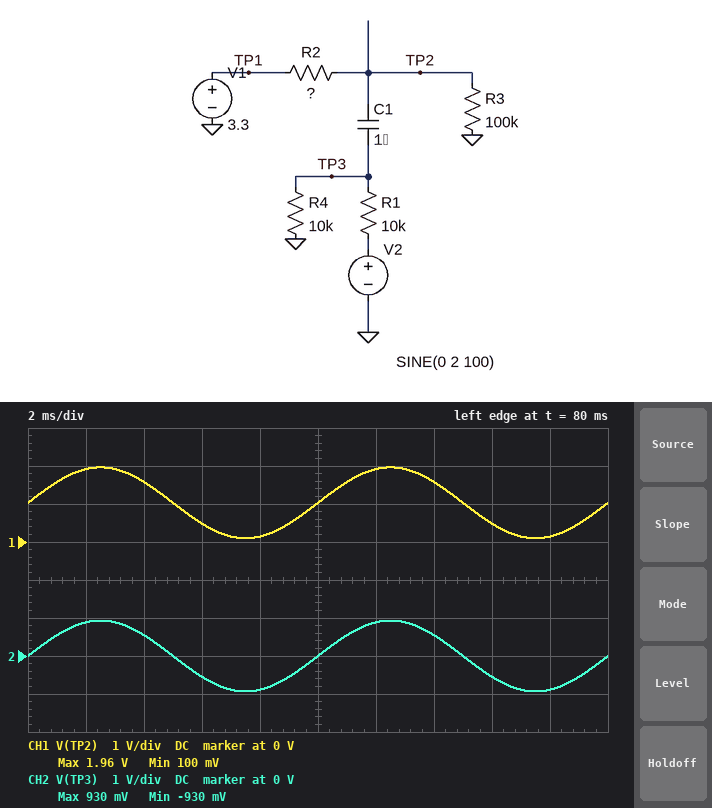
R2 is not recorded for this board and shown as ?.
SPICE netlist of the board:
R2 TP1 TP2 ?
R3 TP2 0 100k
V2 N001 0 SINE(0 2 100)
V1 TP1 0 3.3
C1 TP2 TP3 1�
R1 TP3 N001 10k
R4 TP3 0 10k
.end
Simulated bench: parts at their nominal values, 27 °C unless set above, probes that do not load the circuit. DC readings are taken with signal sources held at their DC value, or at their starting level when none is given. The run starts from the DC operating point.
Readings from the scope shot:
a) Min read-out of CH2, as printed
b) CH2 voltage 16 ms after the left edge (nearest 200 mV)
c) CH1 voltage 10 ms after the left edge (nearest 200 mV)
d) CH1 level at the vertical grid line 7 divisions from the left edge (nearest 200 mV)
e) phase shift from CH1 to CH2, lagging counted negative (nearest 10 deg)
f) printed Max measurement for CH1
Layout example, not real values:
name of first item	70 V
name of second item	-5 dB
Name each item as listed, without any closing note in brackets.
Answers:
Min read-out of CH2, as printed	-930 mV
CH2 voltage 16 ms after the left edge	-600 mV
CH1 voltage 10 ms after the left edge	1.0 V
CH1 level at the vertical grid line 7 divisions from the left edge	1.6 V
phase shift from CH1 to CH2, lagging counted negative	0 deg
printed Max measurement for CH1	1.96 V
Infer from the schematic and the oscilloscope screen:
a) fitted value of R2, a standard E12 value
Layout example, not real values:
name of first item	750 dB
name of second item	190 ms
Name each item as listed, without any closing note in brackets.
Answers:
fitted value of R2, a standard E12 value	220 kΩ
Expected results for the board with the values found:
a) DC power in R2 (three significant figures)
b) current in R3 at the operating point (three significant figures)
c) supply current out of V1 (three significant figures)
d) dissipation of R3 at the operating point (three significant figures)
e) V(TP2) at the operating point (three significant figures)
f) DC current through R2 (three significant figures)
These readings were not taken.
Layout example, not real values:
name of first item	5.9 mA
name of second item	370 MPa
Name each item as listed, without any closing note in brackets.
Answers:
DC power in R2	23.4 µW
current in R3 at the operating point	10.3 µA
supply current out of V1	10.3 µA
dissipation of R3 at the operating point	10.6 µW
V(TP2) at the operating point	1.03 V
DC current through R2	10.3 µA
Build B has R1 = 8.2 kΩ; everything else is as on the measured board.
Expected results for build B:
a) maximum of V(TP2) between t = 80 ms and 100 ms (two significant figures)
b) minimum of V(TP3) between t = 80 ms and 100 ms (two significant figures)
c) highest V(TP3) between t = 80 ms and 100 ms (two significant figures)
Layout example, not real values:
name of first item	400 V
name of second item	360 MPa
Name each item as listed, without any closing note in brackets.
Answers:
maximum of V(TP2) between t = 80 ms and 100 ms	2.1 V
minimum of V(TP3) between t = 80 ms and 100 ms	-1.0 V
highest V(TP3) between t = 80 ms and 100 ms	1.0 V
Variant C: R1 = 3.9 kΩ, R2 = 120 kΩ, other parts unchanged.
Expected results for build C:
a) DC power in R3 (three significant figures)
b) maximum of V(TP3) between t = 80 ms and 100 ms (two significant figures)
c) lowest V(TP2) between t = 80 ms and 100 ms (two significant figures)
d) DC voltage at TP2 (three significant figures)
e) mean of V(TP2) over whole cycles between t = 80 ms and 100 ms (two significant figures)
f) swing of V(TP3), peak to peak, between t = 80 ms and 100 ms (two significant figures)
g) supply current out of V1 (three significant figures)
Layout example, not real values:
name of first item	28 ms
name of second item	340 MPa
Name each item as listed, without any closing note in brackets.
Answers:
DC power in R3	22.5 µW
maximum of V(TP3) between t = 80 ms and 100 ms	1.4 V
lowest V(TP2) between t = 80 ms and 100 ms	130 mV
DC voltage at TP2	1.50 V
mean of V(TP2) over whole cycles between t = 80 ms and 100 ms	1.5 V
swing of V(TP3), peak to peak, between t = 80 ms and 100 ms	2.7 V
supply current out of V1	15.0 µA
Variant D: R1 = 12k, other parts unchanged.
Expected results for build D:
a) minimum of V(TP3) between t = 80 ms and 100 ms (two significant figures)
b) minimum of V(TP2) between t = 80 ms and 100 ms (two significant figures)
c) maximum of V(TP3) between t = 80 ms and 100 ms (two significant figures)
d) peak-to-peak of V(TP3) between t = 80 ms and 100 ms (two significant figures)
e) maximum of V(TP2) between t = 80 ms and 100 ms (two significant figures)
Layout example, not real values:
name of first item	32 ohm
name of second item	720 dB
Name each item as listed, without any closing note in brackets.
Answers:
minimum of V(TP3) between t = 80 ms and 100 ms	-840 mV
minimum of V(TP2) between t = 80 ms and 100 ms	190 mV
maximum of V(TP3) between t = 80 ms and 100 ms	840 mV
peak-to-peak of V(TP3) between t = 80 ms and 100 ms	1.7 V
maximum of V(TP2) between t = 80 ms and 100 ms	1.9 V
